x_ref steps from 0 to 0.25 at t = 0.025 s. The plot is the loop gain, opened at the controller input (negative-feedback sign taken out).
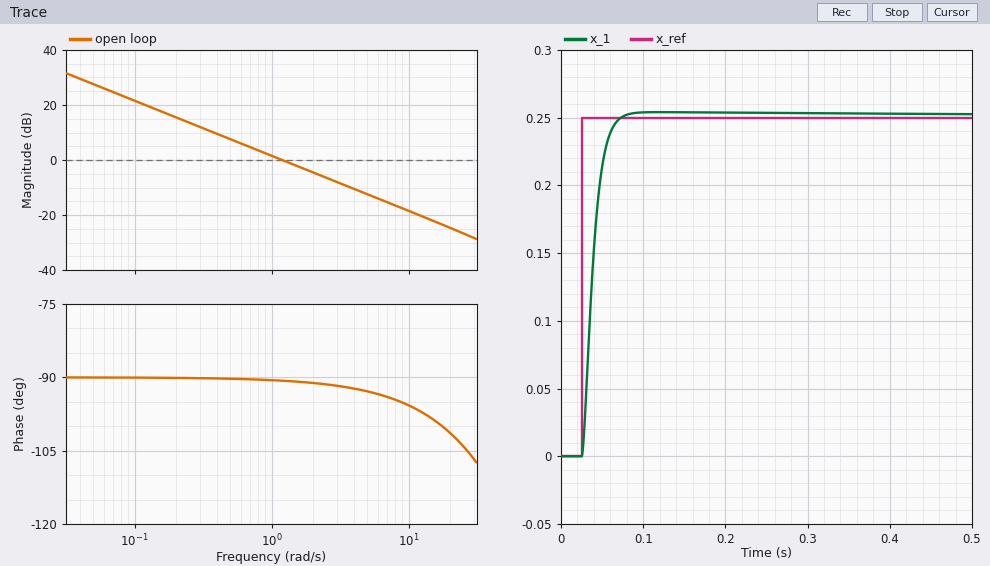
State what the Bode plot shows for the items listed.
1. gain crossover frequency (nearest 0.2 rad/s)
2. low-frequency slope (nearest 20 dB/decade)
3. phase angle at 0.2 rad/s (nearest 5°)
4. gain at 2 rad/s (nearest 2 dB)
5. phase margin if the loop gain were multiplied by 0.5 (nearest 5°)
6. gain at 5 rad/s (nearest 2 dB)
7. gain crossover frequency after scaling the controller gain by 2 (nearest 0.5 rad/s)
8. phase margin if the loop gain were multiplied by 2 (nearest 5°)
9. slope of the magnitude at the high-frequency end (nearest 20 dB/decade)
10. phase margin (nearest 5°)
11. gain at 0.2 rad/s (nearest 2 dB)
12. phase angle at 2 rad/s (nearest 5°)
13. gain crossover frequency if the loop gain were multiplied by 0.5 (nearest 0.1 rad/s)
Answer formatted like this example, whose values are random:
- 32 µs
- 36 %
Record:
- 1.2 rad/s
- -20 dB/decade
- -90°
- -4 dB
- 90°
- -12 dB
- 2.5 rad/s
- 90°
- -20 dB/decade
- 90°
- 16 dB
- -90°
- 0.6 rad/s
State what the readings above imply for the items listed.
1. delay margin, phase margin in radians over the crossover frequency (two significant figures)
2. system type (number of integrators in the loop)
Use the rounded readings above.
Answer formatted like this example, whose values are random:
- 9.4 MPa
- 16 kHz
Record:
- 1.3 s
- 1
